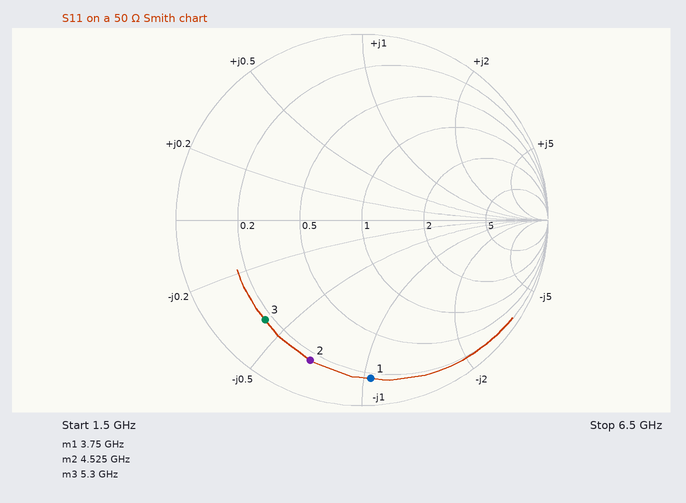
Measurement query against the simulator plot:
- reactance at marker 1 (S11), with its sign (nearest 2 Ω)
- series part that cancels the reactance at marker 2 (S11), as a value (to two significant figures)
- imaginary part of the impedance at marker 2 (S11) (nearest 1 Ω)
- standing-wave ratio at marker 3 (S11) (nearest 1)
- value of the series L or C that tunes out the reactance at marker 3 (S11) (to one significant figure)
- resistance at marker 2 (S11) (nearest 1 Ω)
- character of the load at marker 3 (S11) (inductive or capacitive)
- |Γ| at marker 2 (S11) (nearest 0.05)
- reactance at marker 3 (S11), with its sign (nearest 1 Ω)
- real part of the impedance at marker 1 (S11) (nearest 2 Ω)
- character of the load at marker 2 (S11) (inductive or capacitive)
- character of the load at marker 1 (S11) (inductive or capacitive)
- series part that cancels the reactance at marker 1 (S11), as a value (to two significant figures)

-52 Ω
1.2 nH
-34 Ω
7
600 pH
8 Ω
capacitive
0.80
-21 Ω
8 Ω
capacitive
capacitive
2.2 nH
